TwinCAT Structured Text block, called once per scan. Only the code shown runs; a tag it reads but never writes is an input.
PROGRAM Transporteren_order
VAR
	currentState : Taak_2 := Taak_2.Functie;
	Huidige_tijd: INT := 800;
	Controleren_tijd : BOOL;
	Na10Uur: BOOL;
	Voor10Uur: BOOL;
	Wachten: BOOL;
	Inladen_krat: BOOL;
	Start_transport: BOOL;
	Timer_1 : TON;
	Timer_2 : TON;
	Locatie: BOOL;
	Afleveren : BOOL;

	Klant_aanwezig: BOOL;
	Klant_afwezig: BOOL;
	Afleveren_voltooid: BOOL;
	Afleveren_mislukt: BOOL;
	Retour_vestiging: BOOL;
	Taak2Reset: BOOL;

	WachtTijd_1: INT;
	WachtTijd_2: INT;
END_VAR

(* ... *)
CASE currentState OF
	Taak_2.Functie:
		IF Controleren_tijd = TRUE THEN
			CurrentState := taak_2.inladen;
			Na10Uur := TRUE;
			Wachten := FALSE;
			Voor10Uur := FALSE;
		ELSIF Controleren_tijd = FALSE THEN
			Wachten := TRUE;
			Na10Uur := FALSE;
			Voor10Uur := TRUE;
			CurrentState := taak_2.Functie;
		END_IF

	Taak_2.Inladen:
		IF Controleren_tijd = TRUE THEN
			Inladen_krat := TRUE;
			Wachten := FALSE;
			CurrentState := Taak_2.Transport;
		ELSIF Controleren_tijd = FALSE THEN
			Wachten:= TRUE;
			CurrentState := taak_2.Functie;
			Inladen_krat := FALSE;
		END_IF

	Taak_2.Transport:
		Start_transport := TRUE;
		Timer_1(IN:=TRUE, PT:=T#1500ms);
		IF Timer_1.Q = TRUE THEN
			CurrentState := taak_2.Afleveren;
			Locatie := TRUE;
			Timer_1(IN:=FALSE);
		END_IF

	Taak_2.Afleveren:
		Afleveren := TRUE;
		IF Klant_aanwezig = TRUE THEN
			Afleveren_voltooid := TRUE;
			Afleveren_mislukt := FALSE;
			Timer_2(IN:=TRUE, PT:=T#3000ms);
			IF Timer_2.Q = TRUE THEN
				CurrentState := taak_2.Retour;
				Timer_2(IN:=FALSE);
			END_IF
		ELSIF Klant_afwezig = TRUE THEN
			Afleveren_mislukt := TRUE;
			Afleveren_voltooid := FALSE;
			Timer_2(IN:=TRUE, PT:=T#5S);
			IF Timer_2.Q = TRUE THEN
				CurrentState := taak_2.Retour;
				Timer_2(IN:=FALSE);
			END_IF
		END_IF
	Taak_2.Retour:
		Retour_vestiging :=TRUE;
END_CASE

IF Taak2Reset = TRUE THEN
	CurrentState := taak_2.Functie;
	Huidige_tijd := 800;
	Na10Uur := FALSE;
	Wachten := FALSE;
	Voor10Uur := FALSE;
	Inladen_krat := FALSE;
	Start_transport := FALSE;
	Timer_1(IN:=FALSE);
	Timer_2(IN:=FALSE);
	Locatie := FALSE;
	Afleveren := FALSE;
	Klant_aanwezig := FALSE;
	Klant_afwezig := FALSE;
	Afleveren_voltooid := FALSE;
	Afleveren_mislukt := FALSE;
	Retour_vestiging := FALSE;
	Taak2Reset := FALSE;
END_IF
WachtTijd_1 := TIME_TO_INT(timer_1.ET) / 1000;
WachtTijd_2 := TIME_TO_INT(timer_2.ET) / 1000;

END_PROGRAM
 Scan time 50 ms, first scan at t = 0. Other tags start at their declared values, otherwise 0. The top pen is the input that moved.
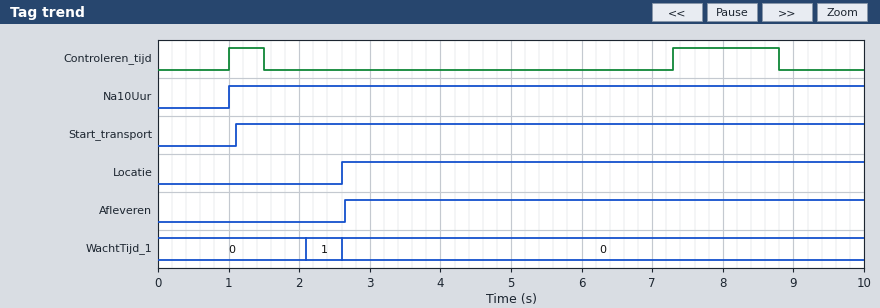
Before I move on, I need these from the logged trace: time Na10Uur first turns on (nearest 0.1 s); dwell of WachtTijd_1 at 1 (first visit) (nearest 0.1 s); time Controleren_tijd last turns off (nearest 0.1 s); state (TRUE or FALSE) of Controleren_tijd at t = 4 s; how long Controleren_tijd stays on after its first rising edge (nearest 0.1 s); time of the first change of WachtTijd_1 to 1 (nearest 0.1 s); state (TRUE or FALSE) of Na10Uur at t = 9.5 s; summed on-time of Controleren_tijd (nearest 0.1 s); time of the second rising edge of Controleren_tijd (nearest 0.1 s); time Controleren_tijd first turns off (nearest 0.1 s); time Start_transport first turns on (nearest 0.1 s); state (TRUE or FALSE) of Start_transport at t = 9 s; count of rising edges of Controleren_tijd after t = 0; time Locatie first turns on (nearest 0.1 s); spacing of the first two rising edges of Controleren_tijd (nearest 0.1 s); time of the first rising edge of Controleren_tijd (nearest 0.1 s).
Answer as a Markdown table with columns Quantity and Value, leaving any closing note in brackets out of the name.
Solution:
| Quantity | Value |
|---|---|
| time Na10Uur first turns on | 1.0 s |
| dwell of WachtTijd_1 at 1 (first visit) | 0.5 s |
| time Controleren_tijd last turns off | 8.8 s |
| state (TRUE or FALSE) of Controleren_tijd at t = 4 s | FALSE |
| how long Controleren_tijd stays on after its first rising edge | 0.5 s |
| time of the first change of WachtTijd_1 to 1 | 2.1 s |
| state (TRUE or FALSE) of Na10Uur at t = 9.5 s | TRUE |
| summed on-time of Controleren_tijd | 2.0 s |
| time of the second rising edge of Controleren_tijd | 7.3 s |
| time Controleren_tijd first turns off | 1.5 s |
| time Start_transport first turns on | 1.1 s |
| state (TRUE or FALSE) of Start_transport at t = 9 s | TRUE |
| count of rising edges of Controleren_tijd after t = 0 | 2 |
| time Locatie first turns on | 2.6 s |
| spacing of the first two rising edges of Controleren_tijd | 6.3 s |
| time of the first rising edge of Controleren_tijd | 1.0 s |
